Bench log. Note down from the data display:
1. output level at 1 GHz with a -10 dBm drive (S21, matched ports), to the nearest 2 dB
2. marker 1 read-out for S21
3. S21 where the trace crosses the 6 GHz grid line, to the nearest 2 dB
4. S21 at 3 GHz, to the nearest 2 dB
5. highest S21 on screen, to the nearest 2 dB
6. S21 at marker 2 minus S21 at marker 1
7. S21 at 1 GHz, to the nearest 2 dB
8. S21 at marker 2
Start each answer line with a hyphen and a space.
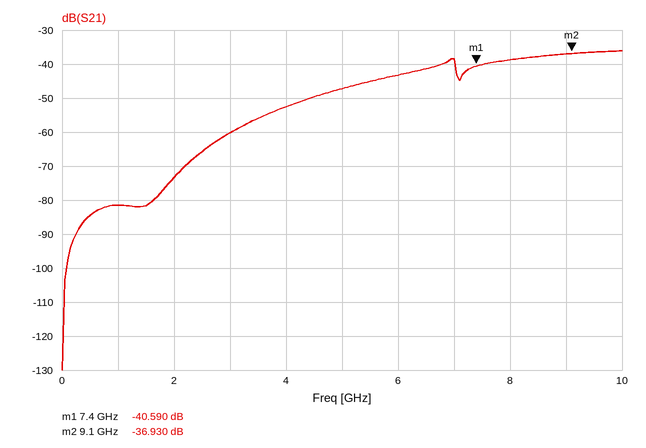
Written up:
- -92 dBm
- -40.590 dB
- -44 dB
- -60 dB
- -36 dB
- 3.660 dB
- -82 dB
- -36.930 dB
